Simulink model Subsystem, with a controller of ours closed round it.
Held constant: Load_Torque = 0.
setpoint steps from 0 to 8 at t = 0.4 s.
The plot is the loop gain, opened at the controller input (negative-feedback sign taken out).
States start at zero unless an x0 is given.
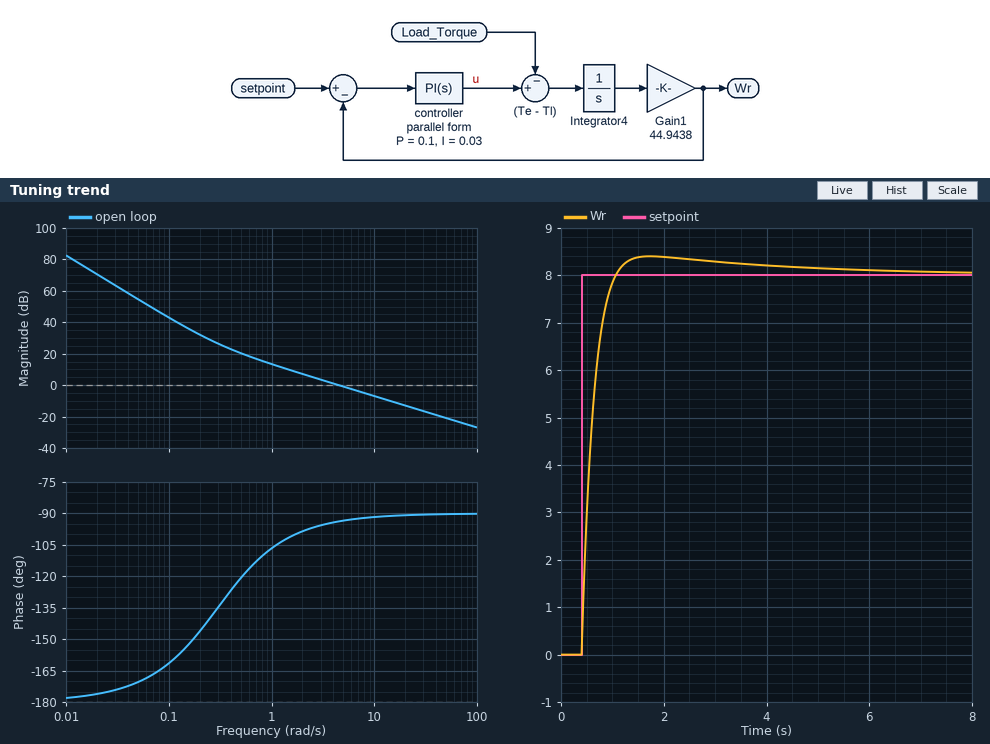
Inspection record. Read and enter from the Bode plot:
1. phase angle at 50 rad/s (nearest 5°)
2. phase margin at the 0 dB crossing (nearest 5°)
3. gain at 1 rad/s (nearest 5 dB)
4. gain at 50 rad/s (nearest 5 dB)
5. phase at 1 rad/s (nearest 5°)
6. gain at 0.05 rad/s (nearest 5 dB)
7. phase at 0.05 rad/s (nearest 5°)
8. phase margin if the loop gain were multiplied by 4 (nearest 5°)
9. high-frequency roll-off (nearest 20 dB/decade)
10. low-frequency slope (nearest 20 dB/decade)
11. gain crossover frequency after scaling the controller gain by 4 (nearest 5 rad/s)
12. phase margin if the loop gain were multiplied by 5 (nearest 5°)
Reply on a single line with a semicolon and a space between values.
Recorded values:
-90°; 85°; 15 dB; -20 dB; -105°; 55 dB; -170°; 90°; -20 dB/decade; -40 dB/decade; 20 rad/s; 90°
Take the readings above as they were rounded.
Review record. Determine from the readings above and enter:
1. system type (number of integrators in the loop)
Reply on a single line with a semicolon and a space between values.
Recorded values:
2
